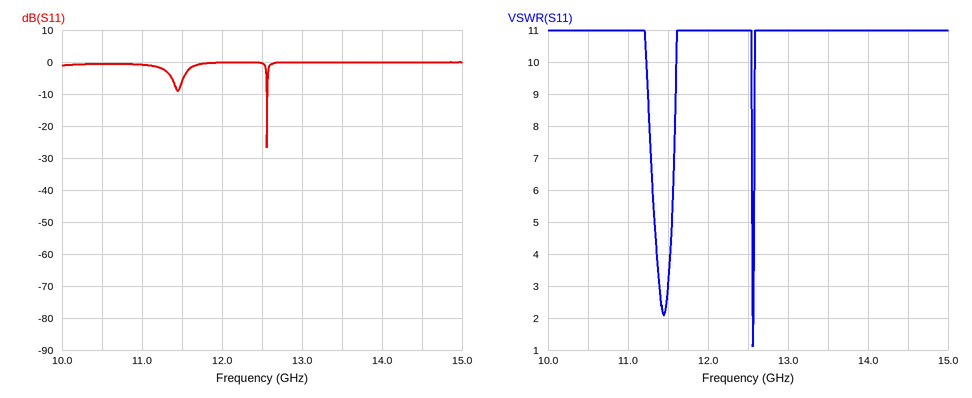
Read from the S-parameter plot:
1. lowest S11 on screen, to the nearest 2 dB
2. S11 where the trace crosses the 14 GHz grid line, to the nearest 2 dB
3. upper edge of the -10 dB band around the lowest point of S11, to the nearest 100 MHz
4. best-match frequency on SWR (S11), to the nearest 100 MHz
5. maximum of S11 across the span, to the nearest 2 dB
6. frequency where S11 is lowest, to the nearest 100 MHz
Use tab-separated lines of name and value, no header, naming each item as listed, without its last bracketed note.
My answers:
lowest S11 on screen, to the nearest 2 dB	-26 dB
S11 where the trace crosses the 14 GHz grid line, to the nearest 2 dB	0 dB
upper edge of the -10 dB band around the lowest point of S11, to the nearest 100 MHz	12.6 GHz
best-match frequency on SWR (S11), to the nearest 100 MHz	12.6 GHz
maximum of S11 across the span, to the nearest 2 dB	0 dB
frequency where S11 is lowest, to the nearest 100 MHz	12.6 GHz
